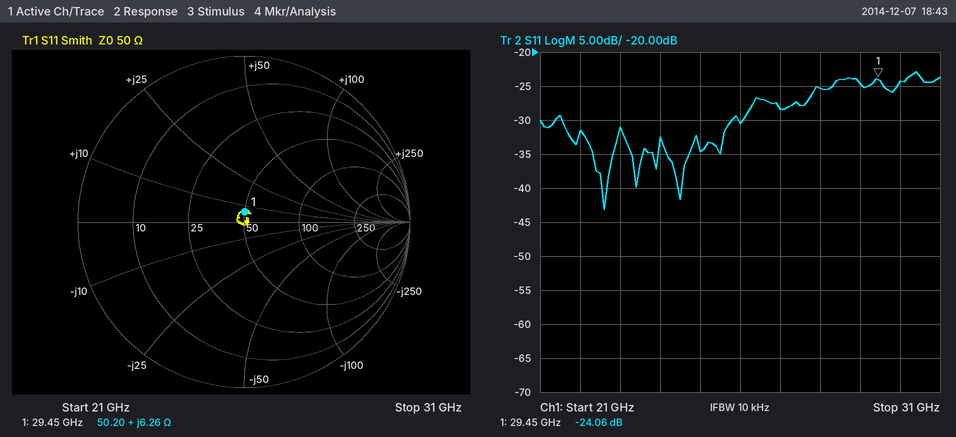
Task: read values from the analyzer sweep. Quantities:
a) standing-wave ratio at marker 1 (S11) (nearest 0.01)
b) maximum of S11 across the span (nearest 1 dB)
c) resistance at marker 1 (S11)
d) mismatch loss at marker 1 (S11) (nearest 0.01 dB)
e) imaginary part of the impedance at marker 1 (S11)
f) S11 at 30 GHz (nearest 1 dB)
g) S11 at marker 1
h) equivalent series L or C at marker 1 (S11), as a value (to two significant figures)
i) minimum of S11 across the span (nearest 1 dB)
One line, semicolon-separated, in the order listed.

1.13; -23 dB; 50.20 Ω; 0.02 dB; +6.26 Ω; -24 dB; -24.06 dB; 34 pH; -43 dB
